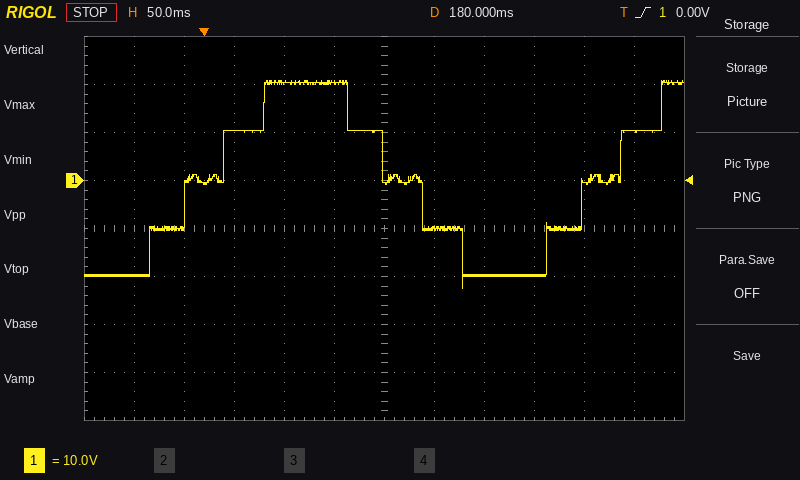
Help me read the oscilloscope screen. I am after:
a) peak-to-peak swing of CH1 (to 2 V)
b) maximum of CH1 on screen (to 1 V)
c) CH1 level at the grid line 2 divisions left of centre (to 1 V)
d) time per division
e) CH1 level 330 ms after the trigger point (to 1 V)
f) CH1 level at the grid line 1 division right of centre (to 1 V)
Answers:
44 V
21 V
20 V
50 ms
-20 V
-10 V
